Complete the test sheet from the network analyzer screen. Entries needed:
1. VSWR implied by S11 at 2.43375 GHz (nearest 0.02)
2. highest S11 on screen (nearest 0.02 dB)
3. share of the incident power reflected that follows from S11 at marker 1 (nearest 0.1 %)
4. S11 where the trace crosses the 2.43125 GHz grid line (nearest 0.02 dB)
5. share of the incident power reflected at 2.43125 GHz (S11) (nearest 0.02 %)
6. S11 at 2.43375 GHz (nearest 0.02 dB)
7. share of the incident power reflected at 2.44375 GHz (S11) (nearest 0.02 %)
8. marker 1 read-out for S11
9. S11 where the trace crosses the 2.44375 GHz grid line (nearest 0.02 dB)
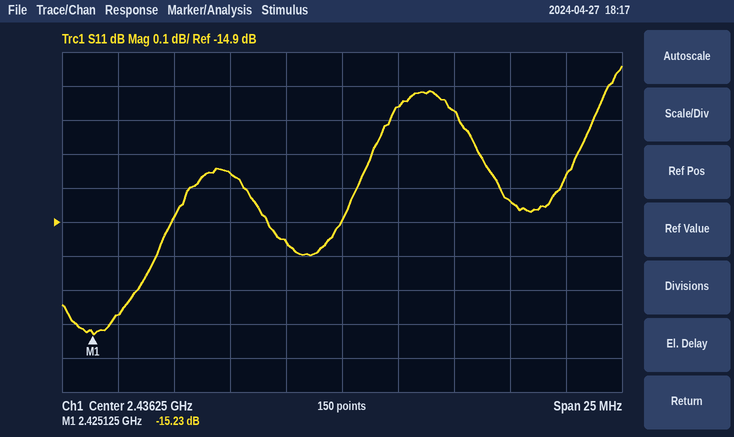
1.44
-14.44 dB
3.0 %
-14.76 dB
3.34 %
-14.96 dB
3.28 %
-15.23 dB
-14.84 dB
